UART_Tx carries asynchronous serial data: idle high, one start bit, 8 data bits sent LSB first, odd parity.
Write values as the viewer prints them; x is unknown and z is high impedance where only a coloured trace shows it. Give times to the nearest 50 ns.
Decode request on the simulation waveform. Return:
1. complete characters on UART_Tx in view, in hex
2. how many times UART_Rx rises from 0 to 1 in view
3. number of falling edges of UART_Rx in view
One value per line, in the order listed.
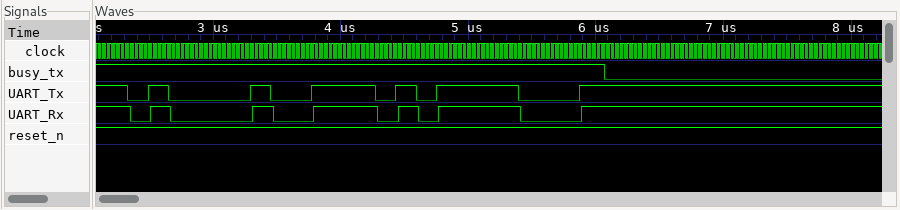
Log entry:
21, 3D
6
6
